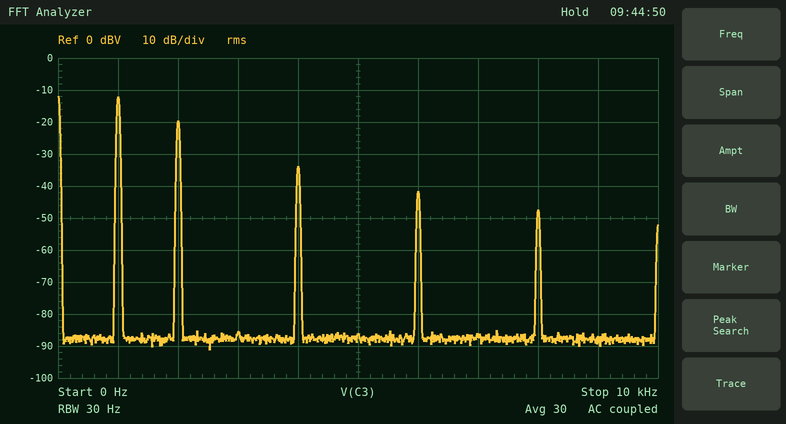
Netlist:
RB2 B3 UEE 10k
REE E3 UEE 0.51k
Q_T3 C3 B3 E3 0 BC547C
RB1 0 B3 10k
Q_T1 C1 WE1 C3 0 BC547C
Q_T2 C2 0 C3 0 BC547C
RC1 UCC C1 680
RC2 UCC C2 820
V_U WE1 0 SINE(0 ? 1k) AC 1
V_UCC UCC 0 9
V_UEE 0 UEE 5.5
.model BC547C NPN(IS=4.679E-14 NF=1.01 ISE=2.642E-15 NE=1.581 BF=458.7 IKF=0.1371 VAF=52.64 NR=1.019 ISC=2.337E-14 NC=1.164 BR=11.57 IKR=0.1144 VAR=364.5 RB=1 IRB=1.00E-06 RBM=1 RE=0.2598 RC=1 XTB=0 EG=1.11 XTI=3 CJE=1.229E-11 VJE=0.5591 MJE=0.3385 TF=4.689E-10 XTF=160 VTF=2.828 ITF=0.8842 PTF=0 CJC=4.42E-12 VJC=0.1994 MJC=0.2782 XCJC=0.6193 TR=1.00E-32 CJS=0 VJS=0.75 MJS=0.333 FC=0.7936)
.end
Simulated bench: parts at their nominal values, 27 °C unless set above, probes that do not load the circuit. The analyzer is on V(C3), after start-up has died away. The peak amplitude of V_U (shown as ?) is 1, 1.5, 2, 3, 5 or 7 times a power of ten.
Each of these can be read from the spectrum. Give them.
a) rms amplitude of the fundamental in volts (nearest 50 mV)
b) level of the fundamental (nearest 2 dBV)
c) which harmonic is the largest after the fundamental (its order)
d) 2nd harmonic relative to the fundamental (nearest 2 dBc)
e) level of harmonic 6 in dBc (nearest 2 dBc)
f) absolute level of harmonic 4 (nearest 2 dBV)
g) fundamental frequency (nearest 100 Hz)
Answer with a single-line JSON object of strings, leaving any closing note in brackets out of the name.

{"rms amplitude of the fundamental in volts": "250 mV", "level of the fundamental": "-12 dBV", "which harmonic is the largest after the fundamental": "2", "2nd harmonic relative to the fundamental": "-8 dBc", "level of harmonic 6 in dBc": "-30 dBc", "absolute level of harmonic 4": "-34 dBV", "fundamental frequency": "1.0 kHz"}
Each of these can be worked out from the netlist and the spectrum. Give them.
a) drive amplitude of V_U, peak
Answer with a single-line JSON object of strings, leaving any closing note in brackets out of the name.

{"drive amplitude of V_U, peak": "700 mV"}
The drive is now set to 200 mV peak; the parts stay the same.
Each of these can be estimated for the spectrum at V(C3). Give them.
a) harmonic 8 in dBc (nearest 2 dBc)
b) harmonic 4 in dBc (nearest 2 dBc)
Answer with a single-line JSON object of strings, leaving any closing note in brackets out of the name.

{"harmonic 8 in dBc": "-48 dBc", "harmonic 4 in dBc": "-26 dBc"}
